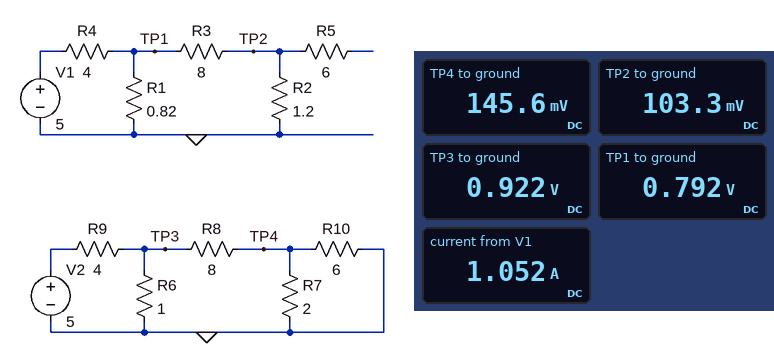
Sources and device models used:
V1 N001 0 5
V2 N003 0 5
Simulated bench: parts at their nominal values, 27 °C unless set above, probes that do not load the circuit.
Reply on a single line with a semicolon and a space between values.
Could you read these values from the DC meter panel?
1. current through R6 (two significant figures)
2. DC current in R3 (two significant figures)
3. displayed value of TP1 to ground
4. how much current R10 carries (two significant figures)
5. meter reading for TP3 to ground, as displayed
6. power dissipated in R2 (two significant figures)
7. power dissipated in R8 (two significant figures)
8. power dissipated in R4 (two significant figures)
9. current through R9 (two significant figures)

920 mA; 86 mA; 0.792 V; 24 mA; 0.922 V; 8.9 mW; 75 mW; 4.4 W; 1.0 A
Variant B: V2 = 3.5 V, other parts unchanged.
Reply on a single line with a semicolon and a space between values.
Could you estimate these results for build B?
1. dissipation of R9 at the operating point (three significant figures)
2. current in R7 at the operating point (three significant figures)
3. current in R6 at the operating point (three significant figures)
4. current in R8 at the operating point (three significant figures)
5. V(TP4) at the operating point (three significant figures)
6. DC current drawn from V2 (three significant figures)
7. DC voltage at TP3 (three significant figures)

2.04 W; 51.0 mA; 646 mA; 68.0 mA; 102 mV; 714 mA; 646 mV
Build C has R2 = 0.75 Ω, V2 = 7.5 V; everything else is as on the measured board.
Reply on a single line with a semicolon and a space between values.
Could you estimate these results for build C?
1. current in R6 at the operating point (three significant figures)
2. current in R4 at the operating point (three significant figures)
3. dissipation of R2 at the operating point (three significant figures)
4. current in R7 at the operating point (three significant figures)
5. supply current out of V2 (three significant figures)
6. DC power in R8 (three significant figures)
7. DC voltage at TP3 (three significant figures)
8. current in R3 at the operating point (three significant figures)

1.38 A; 1.05 A; 6.10 mW; 109 mA; 1.53 A; 170 mW; 1.38 V; 90.2 mA
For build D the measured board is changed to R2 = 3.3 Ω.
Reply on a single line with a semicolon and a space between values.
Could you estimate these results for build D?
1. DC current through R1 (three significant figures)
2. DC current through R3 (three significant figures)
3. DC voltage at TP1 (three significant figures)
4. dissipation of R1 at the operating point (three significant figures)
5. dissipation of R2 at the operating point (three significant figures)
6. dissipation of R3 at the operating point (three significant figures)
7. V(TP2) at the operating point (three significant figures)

978 mA; 71.0 mA; 802 mV; 785 mW; 16.6 mW; 40.3 mW; 234 mV
